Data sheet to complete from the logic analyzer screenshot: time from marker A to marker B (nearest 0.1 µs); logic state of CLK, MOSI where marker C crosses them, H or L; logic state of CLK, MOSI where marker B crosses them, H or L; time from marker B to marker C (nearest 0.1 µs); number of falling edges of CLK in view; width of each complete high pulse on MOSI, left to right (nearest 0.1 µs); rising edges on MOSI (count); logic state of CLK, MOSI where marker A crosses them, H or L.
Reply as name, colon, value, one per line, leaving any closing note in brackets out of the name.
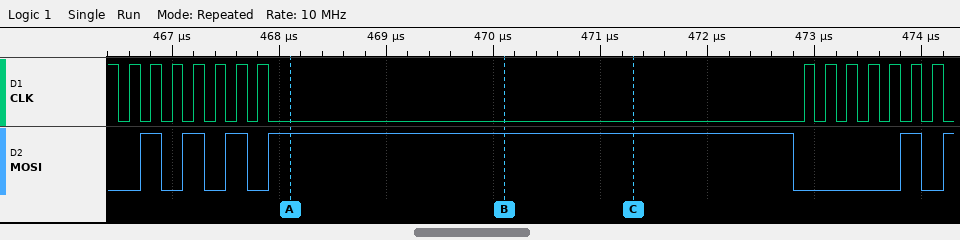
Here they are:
time from marker A to marker B: 2 µs
logic state of CLK, MOSI where marker C crosses them, H or L: CLK=L, MOSI=H
logic state of CLK, MOSI where marker B crosses them, H or L: CLK=L, MOSI=H
time from marker B to marker C: 1.2 µs
number of falling edges of CLK in view: 15
width of each complete high pulse on MOSI, left to right: 0.2 µs, 0.2 µs, 0.2 µs, 4.9 µs, 0.2 µs
rising edges on MOSI: 6
logic state of CLK, MOSI where marker A crosses them, H or L: CLK=L, MOSI=H
